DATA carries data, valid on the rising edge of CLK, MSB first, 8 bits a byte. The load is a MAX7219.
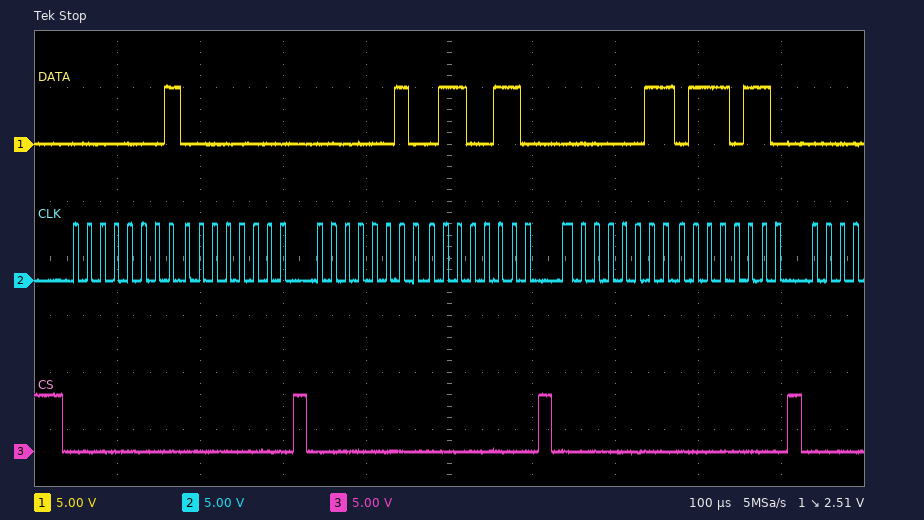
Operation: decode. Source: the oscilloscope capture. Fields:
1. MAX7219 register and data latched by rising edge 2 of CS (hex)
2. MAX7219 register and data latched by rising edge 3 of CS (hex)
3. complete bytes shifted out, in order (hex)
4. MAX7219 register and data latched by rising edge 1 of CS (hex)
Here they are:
register 0x2, data 0x66
register 0x3, data 0x76
01 00 02 66 03 76
register 0x1, data 0x00
